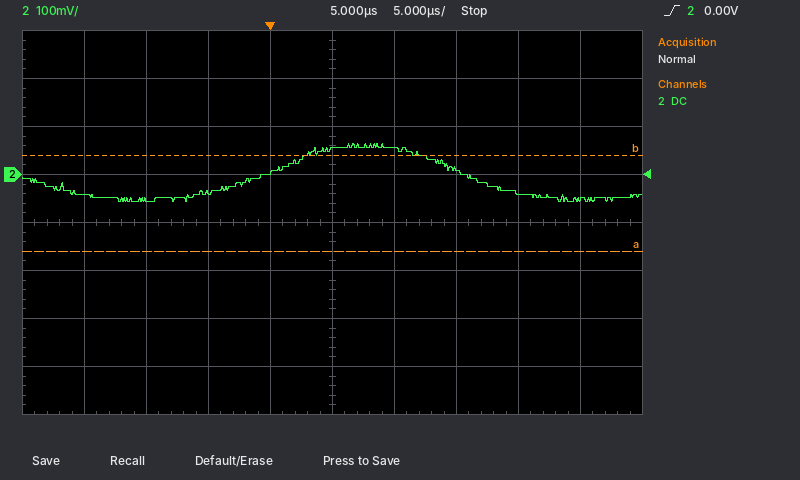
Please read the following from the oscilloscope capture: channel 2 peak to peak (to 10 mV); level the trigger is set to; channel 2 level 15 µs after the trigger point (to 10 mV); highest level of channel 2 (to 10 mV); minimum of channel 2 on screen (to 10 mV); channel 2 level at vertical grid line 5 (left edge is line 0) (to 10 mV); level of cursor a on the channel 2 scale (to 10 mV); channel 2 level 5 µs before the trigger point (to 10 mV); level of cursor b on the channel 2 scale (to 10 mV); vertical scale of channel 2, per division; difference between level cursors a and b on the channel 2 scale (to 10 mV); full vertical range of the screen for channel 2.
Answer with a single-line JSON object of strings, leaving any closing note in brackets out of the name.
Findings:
{"channel 2 peak to peak": "120 mV", "level the trigger is set to": "0.00 V", "channel 2 level 15 µs after the trigger point": "10 mV", "highest level of channel 2": "60 mV", "minimum of channel 2 on screen": "-60 mV", "channel 2 level at vertical grid line 5 (left edge is line 0)": "50 mV", "level of cursor a on the channel 2 scale": "-160 mV", "channel 2 level 5 µs before the trigger point": "-40 mV", "level of cursor b on the channel 2 scale": "40 mV", "vertical scale of channel 2, per division": "100 mV", "difference between level cursors a and b on the channel 2 scale": "200 mV", "full vertical range of the screen for channel 2": "800 mV"}
